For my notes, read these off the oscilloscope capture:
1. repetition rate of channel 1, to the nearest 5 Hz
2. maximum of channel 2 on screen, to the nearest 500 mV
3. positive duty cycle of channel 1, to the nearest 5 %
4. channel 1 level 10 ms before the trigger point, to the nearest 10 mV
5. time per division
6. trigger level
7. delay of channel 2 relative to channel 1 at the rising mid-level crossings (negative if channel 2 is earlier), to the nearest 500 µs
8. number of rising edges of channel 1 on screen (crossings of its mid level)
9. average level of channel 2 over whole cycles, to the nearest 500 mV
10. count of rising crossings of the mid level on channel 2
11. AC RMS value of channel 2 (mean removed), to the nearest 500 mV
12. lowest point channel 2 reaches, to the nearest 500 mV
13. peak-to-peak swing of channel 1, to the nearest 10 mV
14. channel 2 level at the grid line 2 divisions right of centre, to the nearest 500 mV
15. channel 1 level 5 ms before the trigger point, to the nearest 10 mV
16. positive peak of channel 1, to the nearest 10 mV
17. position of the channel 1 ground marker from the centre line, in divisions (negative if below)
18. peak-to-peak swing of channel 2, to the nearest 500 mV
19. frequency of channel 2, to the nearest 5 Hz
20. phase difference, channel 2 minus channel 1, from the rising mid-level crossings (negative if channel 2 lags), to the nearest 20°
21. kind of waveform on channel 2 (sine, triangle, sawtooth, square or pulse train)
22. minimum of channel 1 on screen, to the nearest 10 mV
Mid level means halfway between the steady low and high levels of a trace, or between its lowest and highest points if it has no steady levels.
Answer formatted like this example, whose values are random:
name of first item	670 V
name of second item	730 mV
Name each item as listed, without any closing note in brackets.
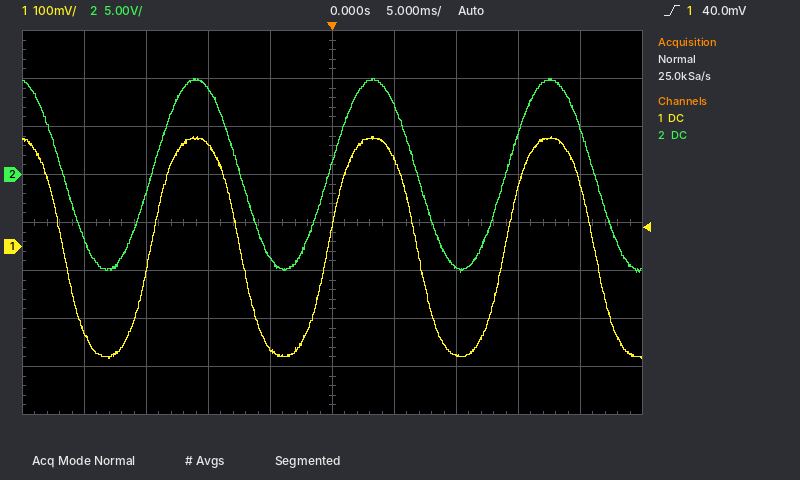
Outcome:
repetition rate of channel 1, to the nearest 5 Hz	70 Hz
maximum of channel 2 on screen, to the nearest 500 mV	10.0 V
positive duty cycle of channel 1, to the nearest 5 %	50 %
channel 1 level 10 ms before the trigger point, to the nearest 10 mV	210 mV
time per division	5 ms
trigger level	40.0 mV
delay of channel 2 relative to channel 1 at the rising mid-level crossings (negative if channel 2 is earlier), to the nearest 500 µs	0.0 ms
number of rising edges of channel 1 on screen	3
average level of channel 2 over whole cycles, to the nearest 500 mV	0.0 V
count of rising crossings of the mid level on channel 2	3
AC RMS value of channel 2 (mean removed), to the nearest 500 mV	7.0 V
lowest point channel 2 reaches, to the nearest 500 mV	-10.0 V
peak-to-peak swing of channel 1, to the nearest 10 mV	460 mV
channel 2 level at the grid line 2 divisions right of centre, to the nearest 500 mV	-9.5 V
channel 1 level 5 ms before the trigger point, to the nearest 10 mV	-210 mV
positive peak of channel 1, to the nearest 10 mV	230 mV
position of the channel 1 ground marker from the centre line, in divisions	-0.5 div
peak-to-peak swing of channel 2, to the nearest 500 mV	20.0 V
frequency of channel 2, to the nearest 5 Hz	70 Hz
phase difference, channel 2 minus channel 1, from the rising mid-level crossings (negative if channel 2 lags), to the nearest 20°	0°
kind of waveform on channel 2	sine
minimum of channel 1 on screen, to the nearest 10 mV	-230 mV
